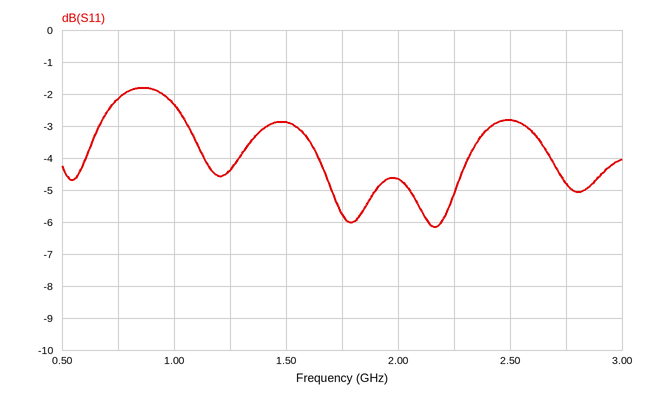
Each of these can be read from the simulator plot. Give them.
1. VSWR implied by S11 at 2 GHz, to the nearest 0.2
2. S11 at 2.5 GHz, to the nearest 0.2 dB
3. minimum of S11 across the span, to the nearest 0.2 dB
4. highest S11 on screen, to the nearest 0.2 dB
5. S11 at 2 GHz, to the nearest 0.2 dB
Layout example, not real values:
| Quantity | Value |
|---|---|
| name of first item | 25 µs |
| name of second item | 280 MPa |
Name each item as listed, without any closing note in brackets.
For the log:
| Quantity | Value |
|---|---|
| VSWR implied by S11 at 2 GHz, to the nearest 0.2 | 3.8 |
| S11 at 2.5 GHz, to the nearest 0.2 dB | -2.8 dB |
| minimum of S11 across the span, to the nearest 0.2 dB | -6.2 dB |
| highest S11 on screen, to the nearest 0.2 dB | -1.8 dB |
| S11 at 2 GHz, to the nearest 0.2 dB | -4.6 dB |
